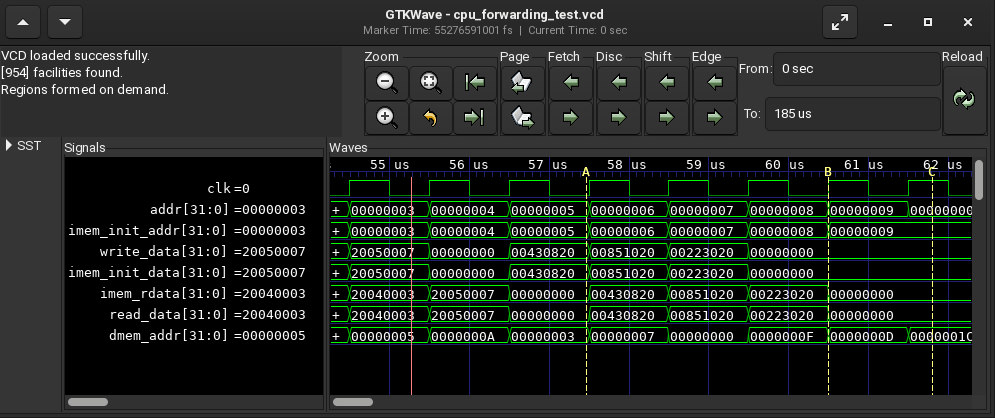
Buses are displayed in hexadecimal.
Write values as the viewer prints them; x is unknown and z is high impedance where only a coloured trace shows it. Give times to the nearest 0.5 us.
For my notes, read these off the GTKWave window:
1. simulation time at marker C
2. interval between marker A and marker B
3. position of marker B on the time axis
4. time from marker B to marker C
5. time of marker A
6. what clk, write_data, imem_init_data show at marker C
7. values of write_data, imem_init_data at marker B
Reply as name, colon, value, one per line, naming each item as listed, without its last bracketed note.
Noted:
simulation time at marker C: 62 us
interval between marker A and marker B: 3 us
position of marker B on the time axis: 60.5 us
time from marker B to marker C: 1.5 us
time of marker A: 57.5 us
what clk, write_data, imem_init_data show at marker C: clk=1, write_data=00000000, imem_init_data=00000000
values of write_data, imem_init_data at marker B: write_data=00000000, imem_init_data=00000000
